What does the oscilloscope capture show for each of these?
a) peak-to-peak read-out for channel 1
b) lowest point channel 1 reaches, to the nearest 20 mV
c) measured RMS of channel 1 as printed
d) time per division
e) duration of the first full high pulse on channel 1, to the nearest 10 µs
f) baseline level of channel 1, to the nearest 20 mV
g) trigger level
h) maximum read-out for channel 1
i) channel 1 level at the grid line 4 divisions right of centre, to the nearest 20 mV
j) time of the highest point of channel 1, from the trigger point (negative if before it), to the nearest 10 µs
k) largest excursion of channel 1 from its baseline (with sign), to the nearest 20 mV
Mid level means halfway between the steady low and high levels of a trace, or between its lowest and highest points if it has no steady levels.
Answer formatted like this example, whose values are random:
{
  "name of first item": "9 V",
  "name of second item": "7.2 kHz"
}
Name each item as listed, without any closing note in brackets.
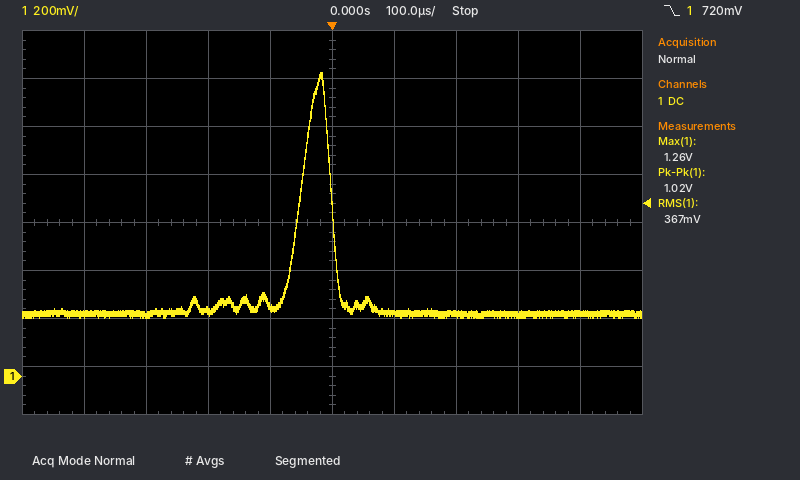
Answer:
{
  "peak-to-peak read-out for channel 1": "1.02 V",
  "lowest point channel 1 reaches, to the nearest 20 mV": "240 mV",
  "measured RMS of channel 1 as printed": "367 mV",
  "time per division": "100 µs",
  "duration of the first full high pulse on channel 1, to the nearest 10 µs": "50 µs",
  "baseline level of channel 1, to the nearest 20 mV": "260 mV",
  "trigger level": "720 mV",
  "maximum read-out for channel 1": "1.26 V",
  "channel 1 level at the grid line 4 divisions right of centre, to the nearest 20 mV": "260 mV",
  "time of the highest point of channel 1, from the trigger point (negative if before it), to the nearest 10 µs": "-20 µs",
  "largest excursion of channel 1 from its baseline (with sign), to the nearest 20 mV": "+1.00 V"
}
